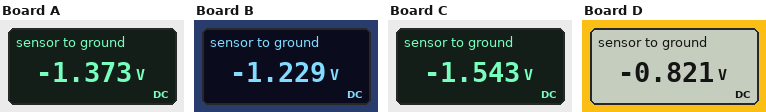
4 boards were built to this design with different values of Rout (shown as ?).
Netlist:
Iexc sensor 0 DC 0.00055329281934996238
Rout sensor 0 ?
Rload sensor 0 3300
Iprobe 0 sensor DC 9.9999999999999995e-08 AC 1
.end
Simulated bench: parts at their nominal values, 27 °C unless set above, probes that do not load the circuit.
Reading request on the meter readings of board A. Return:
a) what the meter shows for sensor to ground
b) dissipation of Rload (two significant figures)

-1.373 V
570 µW
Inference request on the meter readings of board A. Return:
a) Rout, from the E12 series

10 kΩ
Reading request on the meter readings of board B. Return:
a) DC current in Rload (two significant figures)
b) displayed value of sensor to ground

370 µA
-1.229 V
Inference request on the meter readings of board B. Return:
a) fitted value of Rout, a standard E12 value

6.8 kΩ
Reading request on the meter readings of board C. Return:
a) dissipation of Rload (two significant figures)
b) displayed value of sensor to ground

720 µW
-1.543 V
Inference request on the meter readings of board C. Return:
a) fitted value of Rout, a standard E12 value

18 kΩ
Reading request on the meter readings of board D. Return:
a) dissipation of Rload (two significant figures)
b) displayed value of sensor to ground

200 µW
-0.821 V
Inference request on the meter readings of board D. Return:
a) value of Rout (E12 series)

2.7 kΩ
